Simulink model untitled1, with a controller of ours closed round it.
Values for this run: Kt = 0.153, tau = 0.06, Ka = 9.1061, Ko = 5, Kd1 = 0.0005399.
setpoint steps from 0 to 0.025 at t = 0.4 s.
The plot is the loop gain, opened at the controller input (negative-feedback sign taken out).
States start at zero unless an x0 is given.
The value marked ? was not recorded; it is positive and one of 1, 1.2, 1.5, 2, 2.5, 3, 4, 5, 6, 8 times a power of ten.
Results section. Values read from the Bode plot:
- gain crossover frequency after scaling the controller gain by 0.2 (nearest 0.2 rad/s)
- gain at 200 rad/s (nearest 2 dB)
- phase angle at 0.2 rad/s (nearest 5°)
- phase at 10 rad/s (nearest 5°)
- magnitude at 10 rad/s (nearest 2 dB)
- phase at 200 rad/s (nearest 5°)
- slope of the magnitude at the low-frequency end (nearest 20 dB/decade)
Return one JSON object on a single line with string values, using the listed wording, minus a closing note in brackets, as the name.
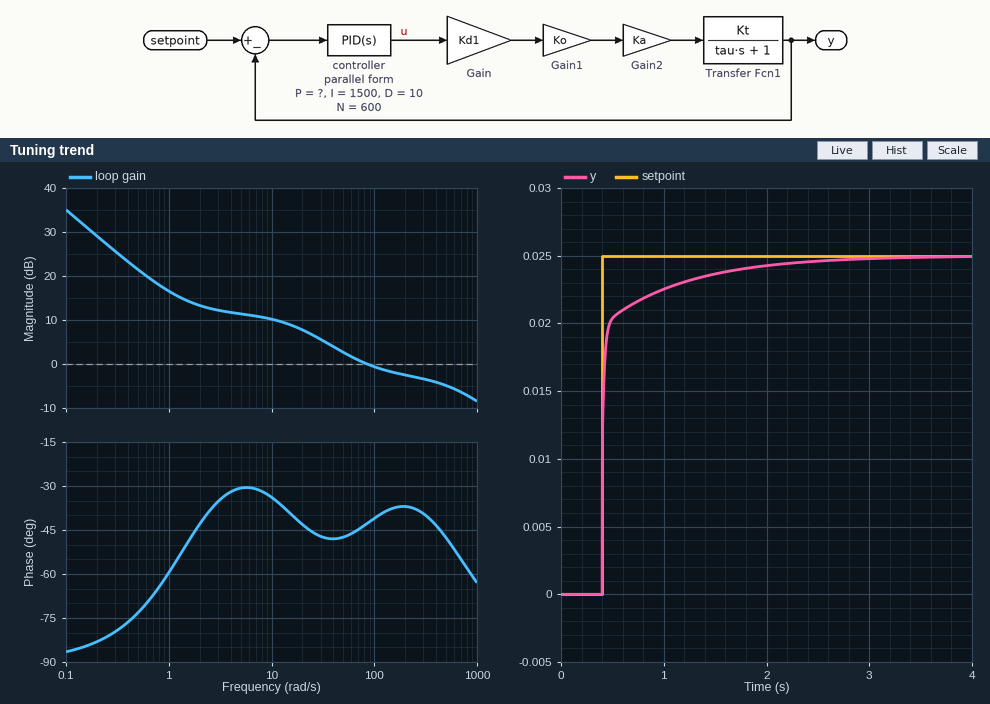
{"gain crossover frequency after scaling the controller gain by 0.2": "1.6 rad/s", "gain at 200 rad/s": "-2 dB", "phase angle at 0.2 rad/s": "-85°", "phase at 10 rad/s": "-35°", "magnitude at 10 rad/s": "10 dB", "phase at 200 rad/s": "-35°", "slope of the magnitude at the low-frequency end": "-20 dB/decade"}
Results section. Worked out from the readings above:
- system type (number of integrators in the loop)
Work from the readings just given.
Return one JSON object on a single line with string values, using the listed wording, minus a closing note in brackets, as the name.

{"system type": "1"}
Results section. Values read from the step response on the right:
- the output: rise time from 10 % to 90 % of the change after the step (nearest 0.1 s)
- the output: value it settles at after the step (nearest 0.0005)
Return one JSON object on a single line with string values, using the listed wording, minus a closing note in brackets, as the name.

{"the output: rise time from 10 % to 90 % of the change after the step": "0.6 s", "the output: value it settles at after the step": "0.0250"}
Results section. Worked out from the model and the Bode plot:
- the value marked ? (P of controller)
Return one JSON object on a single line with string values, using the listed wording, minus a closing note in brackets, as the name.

{"the value marked ?": "1000"}
